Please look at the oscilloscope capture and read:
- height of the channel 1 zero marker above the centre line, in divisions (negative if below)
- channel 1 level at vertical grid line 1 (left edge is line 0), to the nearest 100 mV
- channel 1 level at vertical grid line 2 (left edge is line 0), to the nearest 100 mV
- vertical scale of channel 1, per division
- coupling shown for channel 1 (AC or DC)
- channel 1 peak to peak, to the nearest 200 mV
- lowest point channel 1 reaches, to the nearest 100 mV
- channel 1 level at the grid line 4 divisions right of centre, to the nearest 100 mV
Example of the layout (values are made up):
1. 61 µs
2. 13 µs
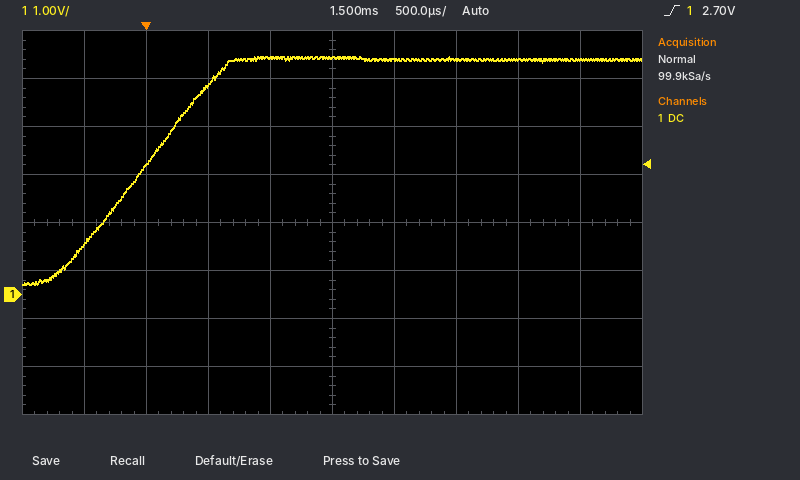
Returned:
1. -1.5 div
2. 1.1 V
3. 2.7 V
4. 1 V
5. DC
6. 4.8 V
7. 200 mV
8. 4.9 V
